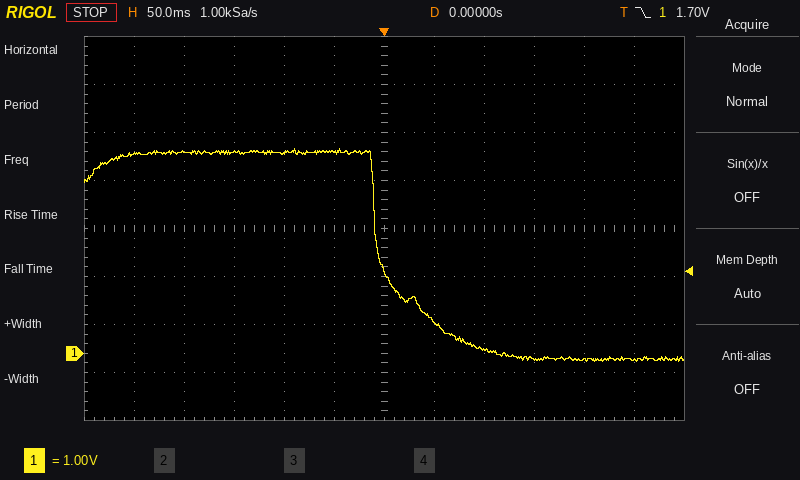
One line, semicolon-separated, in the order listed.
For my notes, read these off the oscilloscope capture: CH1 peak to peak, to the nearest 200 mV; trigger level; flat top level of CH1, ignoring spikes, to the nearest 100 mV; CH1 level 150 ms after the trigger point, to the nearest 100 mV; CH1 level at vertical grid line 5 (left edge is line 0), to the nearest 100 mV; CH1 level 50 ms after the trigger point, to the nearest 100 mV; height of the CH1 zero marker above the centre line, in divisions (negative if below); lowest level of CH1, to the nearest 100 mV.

4.4 V; 1.70 V; 4.2 V; -100 mV; 4.2 V; 700 mV; -2.6 div; -200 mV
